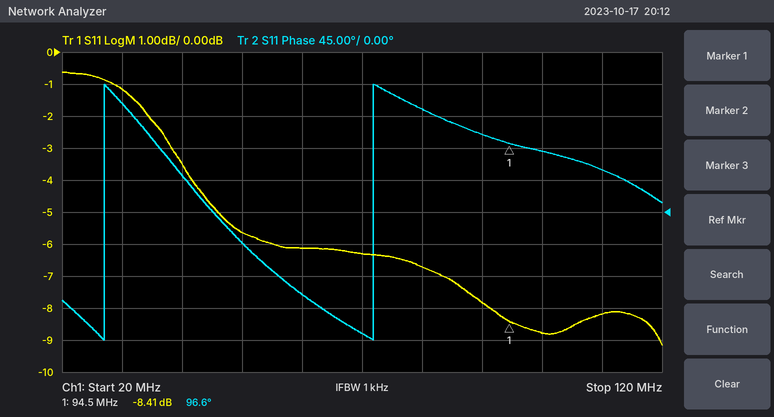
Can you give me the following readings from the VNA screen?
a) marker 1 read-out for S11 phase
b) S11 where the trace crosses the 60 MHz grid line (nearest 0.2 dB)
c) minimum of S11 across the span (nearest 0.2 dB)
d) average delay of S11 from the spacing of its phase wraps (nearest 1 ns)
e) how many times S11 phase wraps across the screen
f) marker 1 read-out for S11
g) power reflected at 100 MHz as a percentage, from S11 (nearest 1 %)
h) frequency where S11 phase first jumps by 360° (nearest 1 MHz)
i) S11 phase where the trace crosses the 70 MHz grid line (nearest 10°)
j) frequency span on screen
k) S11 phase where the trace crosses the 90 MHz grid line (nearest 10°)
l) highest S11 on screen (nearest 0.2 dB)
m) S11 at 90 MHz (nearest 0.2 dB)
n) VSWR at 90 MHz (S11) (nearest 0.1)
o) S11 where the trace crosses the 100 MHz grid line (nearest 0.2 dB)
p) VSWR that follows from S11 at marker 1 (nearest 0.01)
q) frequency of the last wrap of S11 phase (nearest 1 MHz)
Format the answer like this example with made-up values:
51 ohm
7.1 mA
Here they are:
96.6°
-6.2 dB
-9.2 dB
22 ns
2
-8.41 dB
13 %
27 MHz
-170°
100 MHz
110°
-0.6 dB
-7.8 dB
2.4
-8.8 dB
2.22
72 MHz
